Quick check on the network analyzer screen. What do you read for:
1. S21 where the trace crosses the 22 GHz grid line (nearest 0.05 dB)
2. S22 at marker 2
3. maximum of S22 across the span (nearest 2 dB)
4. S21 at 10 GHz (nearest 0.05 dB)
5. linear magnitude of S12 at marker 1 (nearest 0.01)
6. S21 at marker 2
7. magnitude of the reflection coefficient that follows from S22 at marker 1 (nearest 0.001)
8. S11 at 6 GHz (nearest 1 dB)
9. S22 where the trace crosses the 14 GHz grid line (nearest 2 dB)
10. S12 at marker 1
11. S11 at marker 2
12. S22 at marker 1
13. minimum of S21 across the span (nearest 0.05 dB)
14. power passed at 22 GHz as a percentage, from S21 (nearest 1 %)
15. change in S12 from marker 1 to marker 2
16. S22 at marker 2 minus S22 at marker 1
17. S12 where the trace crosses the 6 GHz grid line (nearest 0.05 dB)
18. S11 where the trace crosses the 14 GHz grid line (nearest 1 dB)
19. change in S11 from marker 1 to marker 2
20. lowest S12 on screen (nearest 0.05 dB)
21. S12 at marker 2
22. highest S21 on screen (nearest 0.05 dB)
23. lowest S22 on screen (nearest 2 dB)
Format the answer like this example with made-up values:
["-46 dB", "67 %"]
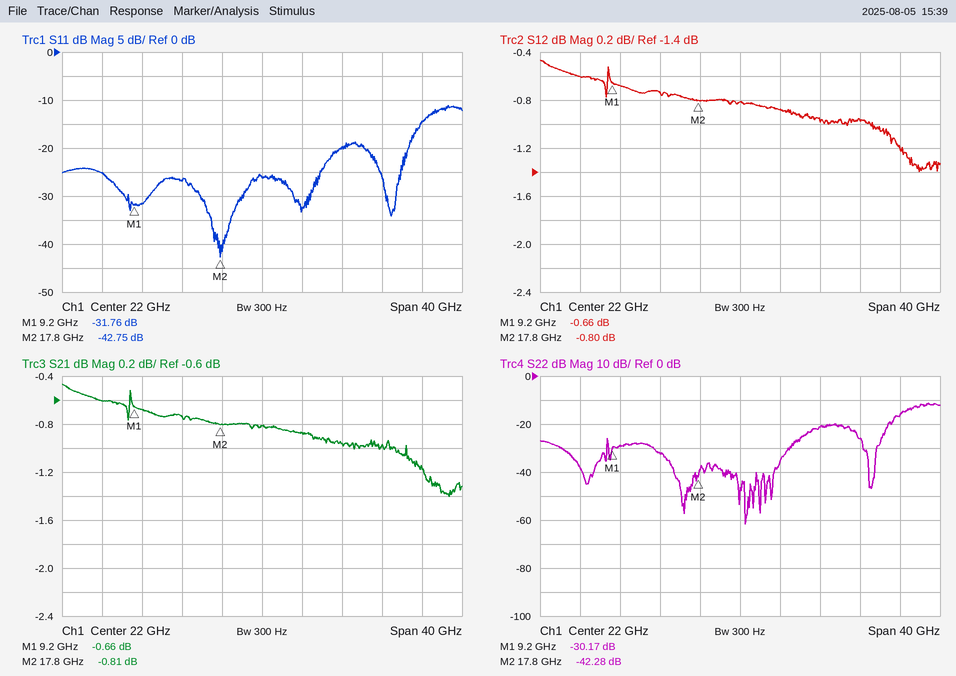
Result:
["-0.80 dB", "-42.28 dB", "-12 dB", "-0.70 dB", "0.93", "-0.81 dB", "0.031", "-25 dB", "-32 dB", "-0.66 dB", "-42.75 dB", "-30.17 dB", "-1.40 dB", "83 %", "-0.14 dB", "-12.11 dB", "-0.60 dB", "-27 dB", "-10.99 dB", "-1.40 dB", "-0.80 dB", "-0.45 dB", "-62 dB"]
